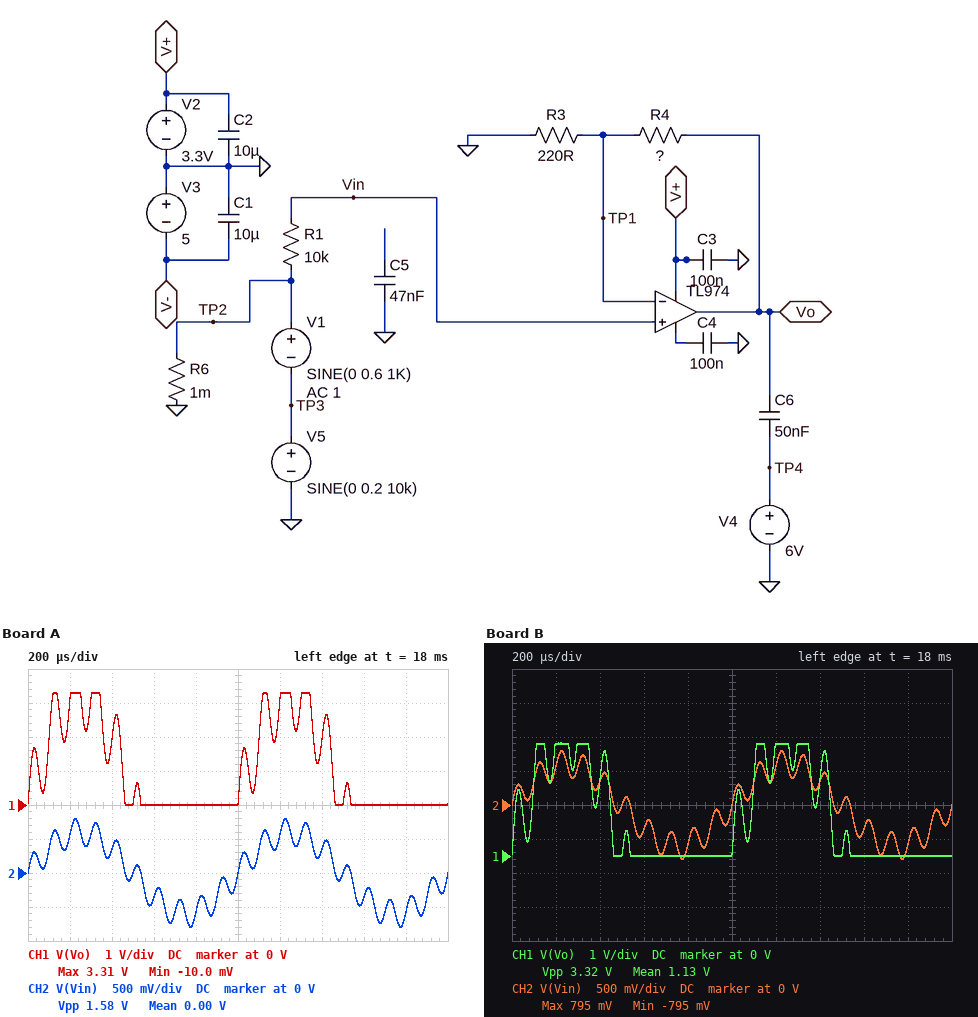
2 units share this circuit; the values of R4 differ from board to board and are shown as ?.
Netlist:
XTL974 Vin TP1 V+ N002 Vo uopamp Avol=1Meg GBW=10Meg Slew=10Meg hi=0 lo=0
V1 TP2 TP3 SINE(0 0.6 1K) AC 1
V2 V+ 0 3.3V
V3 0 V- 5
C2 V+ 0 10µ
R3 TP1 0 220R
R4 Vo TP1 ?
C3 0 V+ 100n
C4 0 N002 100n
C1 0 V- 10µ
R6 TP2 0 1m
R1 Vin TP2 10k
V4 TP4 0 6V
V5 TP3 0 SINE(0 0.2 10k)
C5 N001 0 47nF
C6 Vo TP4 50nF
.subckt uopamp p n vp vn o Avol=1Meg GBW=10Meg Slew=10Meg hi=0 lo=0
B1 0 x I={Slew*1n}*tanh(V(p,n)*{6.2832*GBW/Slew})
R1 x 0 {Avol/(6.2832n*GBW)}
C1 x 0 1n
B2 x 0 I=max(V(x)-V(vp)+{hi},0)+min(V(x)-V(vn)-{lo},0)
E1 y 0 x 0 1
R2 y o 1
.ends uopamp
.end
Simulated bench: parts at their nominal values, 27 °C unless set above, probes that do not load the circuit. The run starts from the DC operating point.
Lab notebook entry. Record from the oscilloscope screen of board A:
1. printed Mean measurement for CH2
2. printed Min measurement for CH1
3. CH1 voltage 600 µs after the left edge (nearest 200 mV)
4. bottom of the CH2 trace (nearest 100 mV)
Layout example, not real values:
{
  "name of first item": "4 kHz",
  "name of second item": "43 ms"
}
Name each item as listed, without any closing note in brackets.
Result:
{
  "printed Mean measurement for CH2": "0.00 V",
  "printed Min measurement for CH1": "-10.0 mV",
  "CH1 voltage 600 µs after the left edge": "0 V",
  "bottom of the CH2 trace": "-800 mV"
}
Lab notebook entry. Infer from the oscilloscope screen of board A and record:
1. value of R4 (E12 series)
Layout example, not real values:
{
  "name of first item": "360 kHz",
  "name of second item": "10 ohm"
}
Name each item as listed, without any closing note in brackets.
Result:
{
  "value of R4": "1 kΩ"
}
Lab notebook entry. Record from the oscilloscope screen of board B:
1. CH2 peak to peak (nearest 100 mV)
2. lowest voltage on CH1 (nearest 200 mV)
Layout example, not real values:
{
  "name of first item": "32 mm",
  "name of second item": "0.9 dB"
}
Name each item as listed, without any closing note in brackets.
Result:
{
  "CH2 peak to peak": "1.6 V",
  "lowest voltage on CH1": "0 V"
}
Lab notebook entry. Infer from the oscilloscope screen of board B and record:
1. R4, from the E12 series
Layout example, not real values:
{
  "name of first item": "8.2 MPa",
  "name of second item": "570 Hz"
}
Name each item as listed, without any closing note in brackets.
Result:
{
  "R4, from the E12 series": "1.2 kΩ"
}
